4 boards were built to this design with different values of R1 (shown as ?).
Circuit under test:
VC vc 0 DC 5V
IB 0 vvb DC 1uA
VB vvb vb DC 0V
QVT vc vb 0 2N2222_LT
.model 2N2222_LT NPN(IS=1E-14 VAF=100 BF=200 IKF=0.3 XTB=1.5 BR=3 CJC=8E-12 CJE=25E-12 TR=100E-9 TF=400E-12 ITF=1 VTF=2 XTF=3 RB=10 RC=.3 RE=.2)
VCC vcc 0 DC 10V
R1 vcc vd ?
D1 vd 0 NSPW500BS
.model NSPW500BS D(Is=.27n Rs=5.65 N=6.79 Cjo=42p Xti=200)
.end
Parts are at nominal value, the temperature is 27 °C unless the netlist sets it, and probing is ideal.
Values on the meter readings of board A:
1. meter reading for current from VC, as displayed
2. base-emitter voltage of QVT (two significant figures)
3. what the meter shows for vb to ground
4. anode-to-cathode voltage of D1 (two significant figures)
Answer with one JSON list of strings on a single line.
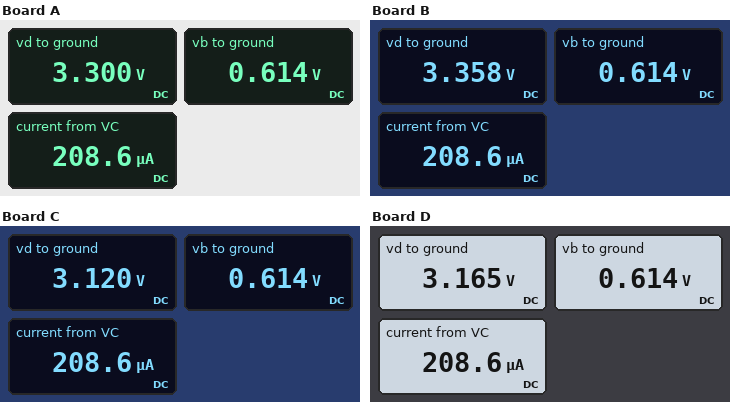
["208.6 µA", "610 mV", "0.614 V", "3.3 V"]
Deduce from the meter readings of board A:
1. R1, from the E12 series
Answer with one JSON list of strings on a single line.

["330 Ω"]
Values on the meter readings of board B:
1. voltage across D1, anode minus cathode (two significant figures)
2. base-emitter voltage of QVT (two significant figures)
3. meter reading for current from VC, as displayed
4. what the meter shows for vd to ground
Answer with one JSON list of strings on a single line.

["3.4 V", "610 mV", "208.6 µA", "3.358 V"]
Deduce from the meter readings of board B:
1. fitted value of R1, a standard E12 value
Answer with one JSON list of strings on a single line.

["270 Ω"]
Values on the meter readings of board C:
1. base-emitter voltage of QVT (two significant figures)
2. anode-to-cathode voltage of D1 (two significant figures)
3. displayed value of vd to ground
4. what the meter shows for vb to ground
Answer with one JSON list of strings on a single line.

["610 mV", "3.1 V", "3.120 V", "0.614 V"]
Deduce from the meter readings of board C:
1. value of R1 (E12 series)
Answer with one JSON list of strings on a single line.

["680 Ω"]
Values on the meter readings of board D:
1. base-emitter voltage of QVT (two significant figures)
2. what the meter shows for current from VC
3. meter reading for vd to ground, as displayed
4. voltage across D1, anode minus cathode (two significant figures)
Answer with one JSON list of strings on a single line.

["610 mV", "208.6 µA", "3.165 V", "3.2 V"]
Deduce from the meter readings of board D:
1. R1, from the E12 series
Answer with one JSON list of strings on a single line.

["560 Ω"]
